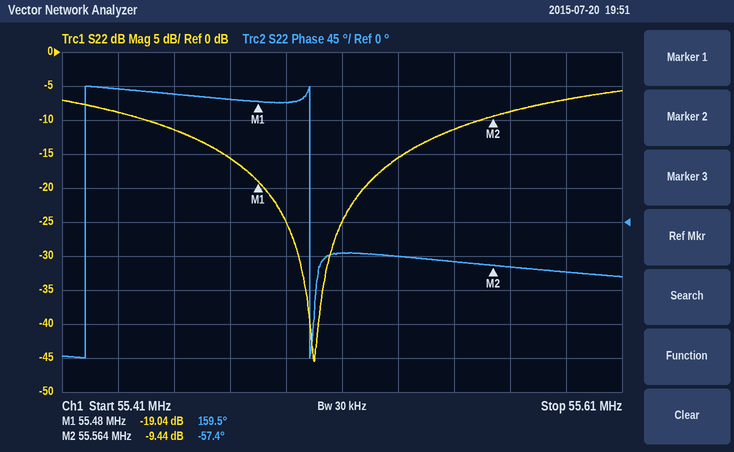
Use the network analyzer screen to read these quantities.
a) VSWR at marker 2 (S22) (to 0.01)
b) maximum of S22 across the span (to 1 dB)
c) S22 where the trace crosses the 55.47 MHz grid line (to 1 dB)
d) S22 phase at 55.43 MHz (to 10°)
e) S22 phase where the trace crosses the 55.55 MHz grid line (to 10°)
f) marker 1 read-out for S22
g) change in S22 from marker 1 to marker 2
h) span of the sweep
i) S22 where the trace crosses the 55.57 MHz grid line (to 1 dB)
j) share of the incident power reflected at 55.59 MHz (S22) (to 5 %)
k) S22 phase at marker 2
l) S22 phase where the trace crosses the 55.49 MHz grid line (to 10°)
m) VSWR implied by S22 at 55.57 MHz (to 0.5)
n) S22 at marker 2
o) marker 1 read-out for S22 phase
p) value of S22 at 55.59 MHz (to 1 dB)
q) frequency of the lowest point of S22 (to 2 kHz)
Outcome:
2.02
-6 dB
-16 dB
180°
-50°
-19.04 dB
9.60 dB
200 kHz
-9 dB
20 %
-57.4°
160°
2.0
-9.44 dB
159.5°
-7 dB
55.500 MHz
